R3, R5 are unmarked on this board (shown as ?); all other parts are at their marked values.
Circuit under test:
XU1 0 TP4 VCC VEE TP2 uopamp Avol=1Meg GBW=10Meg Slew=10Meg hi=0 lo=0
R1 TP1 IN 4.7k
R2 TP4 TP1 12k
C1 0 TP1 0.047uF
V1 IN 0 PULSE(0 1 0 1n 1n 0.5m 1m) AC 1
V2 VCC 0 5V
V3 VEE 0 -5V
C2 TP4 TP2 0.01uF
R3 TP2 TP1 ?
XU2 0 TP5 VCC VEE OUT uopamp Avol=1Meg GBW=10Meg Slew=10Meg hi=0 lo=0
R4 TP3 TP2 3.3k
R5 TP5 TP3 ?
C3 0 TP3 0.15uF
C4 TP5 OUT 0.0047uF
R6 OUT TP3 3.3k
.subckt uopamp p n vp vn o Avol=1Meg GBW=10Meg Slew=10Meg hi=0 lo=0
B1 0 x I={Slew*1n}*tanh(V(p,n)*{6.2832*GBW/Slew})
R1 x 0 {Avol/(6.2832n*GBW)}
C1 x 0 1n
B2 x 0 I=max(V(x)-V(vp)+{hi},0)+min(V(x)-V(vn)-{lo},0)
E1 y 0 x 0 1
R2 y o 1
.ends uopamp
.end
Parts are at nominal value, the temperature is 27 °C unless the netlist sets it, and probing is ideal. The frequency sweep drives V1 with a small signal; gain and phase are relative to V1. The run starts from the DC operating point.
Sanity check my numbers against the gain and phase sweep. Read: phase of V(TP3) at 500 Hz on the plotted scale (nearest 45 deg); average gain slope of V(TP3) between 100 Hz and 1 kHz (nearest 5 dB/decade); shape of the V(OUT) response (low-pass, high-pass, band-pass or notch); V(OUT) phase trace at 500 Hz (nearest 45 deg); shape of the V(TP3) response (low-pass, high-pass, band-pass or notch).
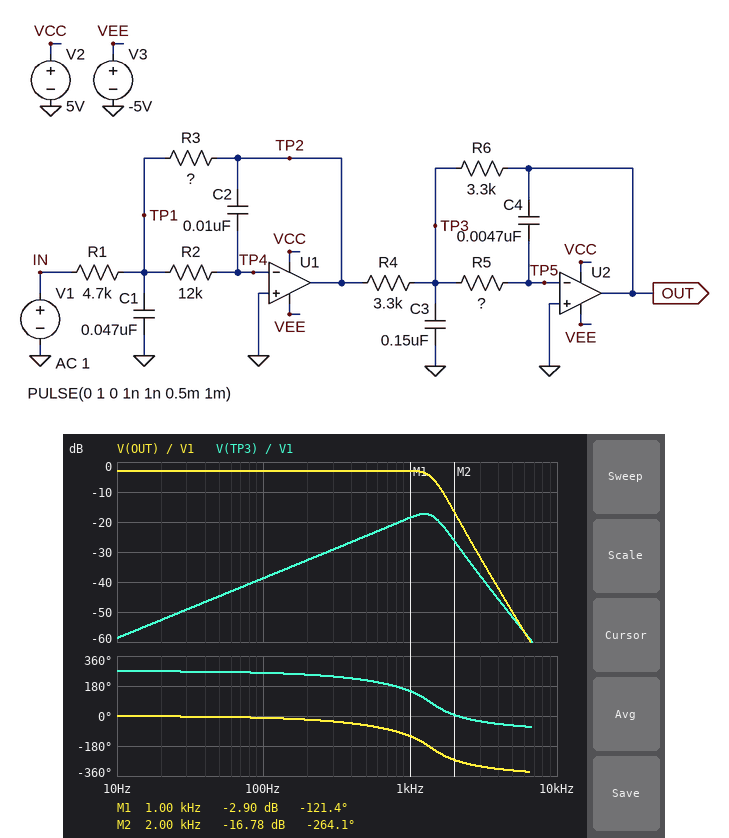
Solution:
225 deg
20 dB/decade
low-pass
-45 deg
band-pass
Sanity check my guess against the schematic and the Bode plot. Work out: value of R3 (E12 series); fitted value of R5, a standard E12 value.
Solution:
3.3 kΩ
5.6 kΩ
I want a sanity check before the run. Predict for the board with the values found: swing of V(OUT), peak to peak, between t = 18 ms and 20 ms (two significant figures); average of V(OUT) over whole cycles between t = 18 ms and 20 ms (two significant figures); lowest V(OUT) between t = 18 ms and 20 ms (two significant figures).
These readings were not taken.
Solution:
910 mV
350 mV
-100 mV
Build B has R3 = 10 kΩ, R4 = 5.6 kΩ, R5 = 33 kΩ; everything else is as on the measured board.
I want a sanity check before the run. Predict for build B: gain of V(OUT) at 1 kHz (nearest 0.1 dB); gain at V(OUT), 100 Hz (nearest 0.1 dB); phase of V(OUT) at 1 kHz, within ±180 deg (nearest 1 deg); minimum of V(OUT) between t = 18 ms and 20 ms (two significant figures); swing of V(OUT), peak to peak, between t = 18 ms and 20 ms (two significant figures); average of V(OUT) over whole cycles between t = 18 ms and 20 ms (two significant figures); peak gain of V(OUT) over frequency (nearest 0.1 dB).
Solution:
-16.6 dB
1.9 dB
107 deg
530 mV
190 mV
630 mV
2.0 dB
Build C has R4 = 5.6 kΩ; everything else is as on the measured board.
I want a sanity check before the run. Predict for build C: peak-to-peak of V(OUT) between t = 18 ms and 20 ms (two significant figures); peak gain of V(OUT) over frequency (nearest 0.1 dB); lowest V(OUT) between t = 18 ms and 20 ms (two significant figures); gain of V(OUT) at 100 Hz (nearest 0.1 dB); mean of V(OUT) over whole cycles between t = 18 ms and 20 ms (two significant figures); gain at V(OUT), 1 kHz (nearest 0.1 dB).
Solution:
570 mV
-6.7 dB
-79 mV
-7.7 dB
210 mV
-6.9 dB
